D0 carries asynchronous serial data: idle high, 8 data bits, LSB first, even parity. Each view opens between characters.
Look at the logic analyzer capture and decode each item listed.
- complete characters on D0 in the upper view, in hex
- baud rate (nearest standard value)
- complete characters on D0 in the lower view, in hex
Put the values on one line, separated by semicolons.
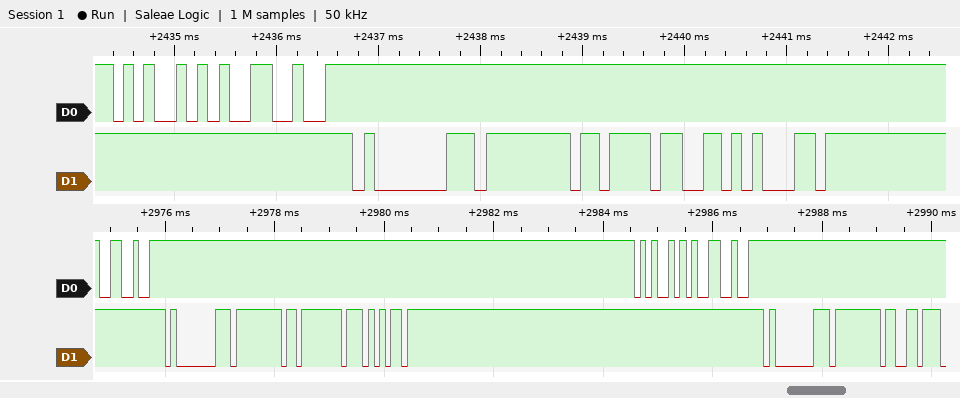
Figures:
A5, 26; 9600 baud; 26, A5, 26
